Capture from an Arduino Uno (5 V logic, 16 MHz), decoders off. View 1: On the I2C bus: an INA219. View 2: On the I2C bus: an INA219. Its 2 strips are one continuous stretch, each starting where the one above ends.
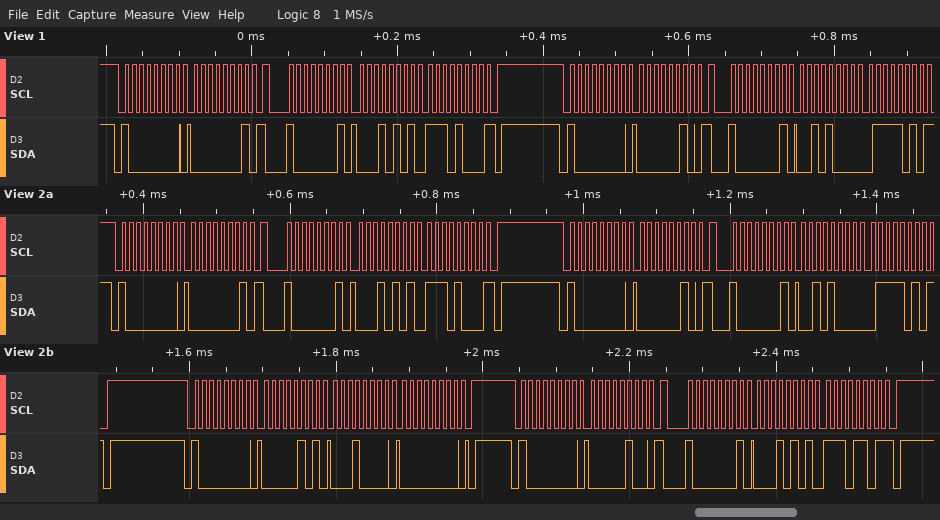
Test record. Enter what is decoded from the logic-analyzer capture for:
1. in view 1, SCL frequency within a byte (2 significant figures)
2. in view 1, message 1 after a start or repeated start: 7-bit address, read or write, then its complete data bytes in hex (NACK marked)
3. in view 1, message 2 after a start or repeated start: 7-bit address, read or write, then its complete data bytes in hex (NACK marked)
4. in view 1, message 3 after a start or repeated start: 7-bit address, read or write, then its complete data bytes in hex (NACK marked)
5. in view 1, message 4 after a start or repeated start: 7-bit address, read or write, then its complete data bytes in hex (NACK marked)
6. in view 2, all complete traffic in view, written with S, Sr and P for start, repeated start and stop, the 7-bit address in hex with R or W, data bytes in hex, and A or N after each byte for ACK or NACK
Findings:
100 kHz
0x40 write: 01
0x40 read: 15 E8 NACK
0x40 write: 02
0x40 read: 28 7A NACK
S 40W A 01 A Sr 40R A 15 A E8 N P S 40W A 02 A Sr 40R A 28 A 7A N P S 40W A 05 A 10 A 00 A P S 40W A 04 A Sr 40R A 15 A ED N P
